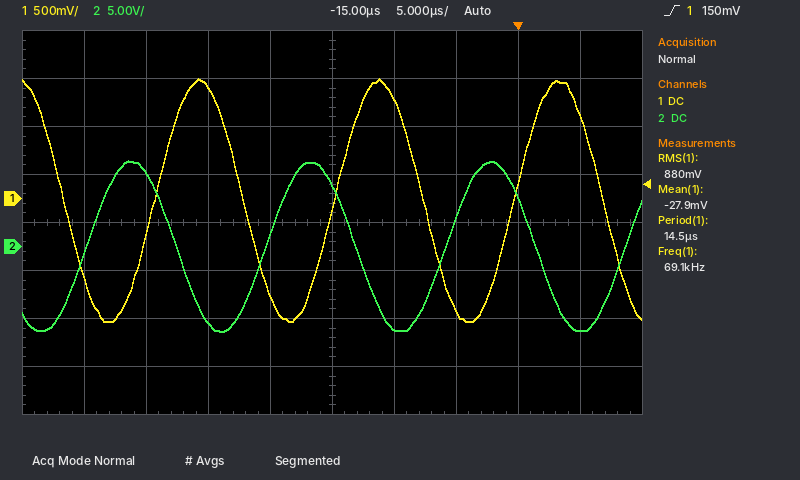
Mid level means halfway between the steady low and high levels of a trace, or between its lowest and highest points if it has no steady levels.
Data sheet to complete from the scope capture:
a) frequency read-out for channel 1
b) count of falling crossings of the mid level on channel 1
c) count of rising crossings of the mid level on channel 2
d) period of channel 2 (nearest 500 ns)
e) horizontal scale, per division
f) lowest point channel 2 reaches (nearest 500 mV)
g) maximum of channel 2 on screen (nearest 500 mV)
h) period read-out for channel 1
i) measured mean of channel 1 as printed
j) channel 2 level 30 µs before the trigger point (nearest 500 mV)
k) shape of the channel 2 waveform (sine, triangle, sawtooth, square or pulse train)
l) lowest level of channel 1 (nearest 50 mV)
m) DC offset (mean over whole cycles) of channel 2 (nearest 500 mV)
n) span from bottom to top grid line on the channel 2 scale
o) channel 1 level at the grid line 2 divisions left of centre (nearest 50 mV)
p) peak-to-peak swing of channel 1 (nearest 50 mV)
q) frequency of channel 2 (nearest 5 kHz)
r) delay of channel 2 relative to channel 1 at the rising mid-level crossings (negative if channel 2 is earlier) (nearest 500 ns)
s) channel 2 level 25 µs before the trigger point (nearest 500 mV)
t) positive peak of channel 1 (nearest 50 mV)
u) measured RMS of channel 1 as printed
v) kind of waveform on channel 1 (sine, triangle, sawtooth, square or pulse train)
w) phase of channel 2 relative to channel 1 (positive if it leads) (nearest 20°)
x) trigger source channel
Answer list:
69.1 kHz
4
4
14.5 µs
5 µs
-9.0 V
9.0 V
14.5 µs
-27.9 mV
7.5 V
sine
-1.30 V
0.0 V
40 V
1.15 V
2.55 V
70 kHz
-5.5 µs
-8.0 V
1.25 V
880 mV
sine
+140°
channel 1
